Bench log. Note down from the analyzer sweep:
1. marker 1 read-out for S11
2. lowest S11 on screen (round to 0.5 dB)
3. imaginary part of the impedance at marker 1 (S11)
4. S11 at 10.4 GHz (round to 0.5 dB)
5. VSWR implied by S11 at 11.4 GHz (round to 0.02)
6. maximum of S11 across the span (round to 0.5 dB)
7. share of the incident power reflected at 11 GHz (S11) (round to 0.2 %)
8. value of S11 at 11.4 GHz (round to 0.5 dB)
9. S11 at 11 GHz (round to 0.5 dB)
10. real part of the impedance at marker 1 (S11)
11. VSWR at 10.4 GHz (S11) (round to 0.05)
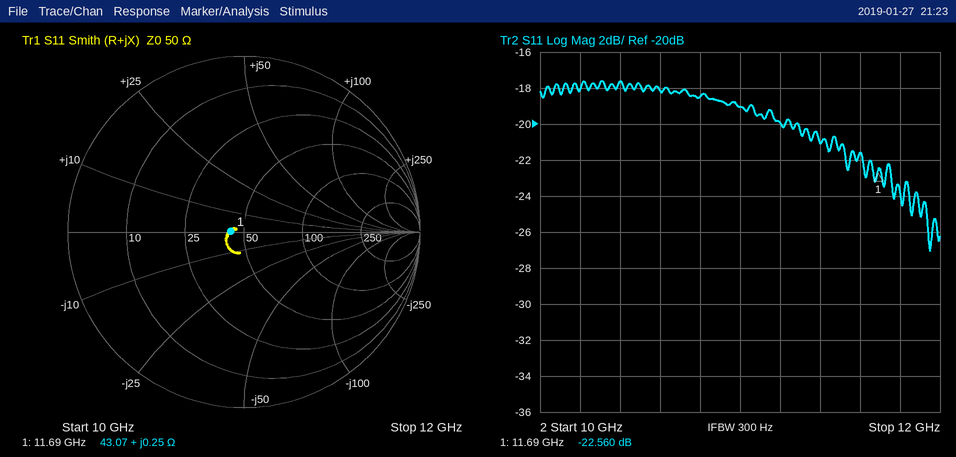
-22.560 dB
-27.0 dB
+0.25 Ω
-17.5 dB
1.20
-17.5 dB
1.2 %
-21.0 dB
-19.0 dB
43.07 Ω
1.30
